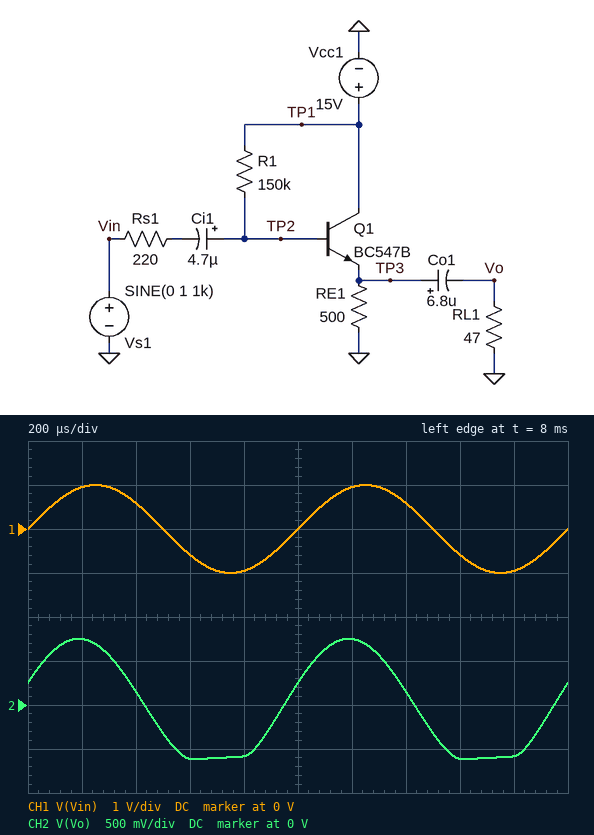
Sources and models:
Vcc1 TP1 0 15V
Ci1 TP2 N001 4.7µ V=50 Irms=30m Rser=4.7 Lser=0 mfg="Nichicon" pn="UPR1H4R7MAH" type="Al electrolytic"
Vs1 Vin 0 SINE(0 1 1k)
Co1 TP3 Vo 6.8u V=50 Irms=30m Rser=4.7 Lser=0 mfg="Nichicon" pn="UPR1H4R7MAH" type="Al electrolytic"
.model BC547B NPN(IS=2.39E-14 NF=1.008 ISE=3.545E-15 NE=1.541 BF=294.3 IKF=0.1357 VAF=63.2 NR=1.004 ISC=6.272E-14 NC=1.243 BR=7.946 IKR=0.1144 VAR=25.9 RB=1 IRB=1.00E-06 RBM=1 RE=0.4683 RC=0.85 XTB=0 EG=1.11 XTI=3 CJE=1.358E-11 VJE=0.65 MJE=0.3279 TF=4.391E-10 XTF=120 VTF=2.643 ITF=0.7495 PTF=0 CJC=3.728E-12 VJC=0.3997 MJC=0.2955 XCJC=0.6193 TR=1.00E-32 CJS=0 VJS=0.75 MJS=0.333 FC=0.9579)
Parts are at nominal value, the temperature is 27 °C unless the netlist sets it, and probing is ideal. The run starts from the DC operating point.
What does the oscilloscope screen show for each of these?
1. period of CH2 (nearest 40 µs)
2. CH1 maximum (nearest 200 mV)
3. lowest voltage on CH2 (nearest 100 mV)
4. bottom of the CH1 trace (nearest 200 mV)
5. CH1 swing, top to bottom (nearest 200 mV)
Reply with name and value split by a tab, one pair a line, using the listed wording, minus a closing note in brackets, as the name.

period of CH2	1.00 ms
CH1 maximum	1.0 V
lowest voltage on CH2	-600 mV
bottom of the CH1 trace	-1.0 V
CH1 swing, top to bottom	2.0 V
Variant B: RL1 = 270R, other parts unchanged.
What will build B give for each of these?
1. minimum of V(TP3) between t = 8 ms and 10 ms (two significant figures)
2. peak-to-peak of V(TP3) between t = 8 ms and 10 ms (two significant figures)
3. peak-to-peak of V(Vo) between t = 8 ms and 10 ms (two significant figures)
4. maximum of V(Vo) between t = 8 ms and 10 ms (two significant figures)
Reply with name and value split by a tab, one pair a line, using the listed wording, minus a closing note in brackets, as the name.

minimum of V(TP3) between t = 8 ms and 10 ms	6.1 V
peak-to-peak of V(TP3) between t = 8 ms and 10 ms	2.0 V
peak-to-peak of V(Vo) between t = 8 ms and 10 ms	1.9 V
maximum of V(Vo) between t = 8 ms and 10 ms	960 mV
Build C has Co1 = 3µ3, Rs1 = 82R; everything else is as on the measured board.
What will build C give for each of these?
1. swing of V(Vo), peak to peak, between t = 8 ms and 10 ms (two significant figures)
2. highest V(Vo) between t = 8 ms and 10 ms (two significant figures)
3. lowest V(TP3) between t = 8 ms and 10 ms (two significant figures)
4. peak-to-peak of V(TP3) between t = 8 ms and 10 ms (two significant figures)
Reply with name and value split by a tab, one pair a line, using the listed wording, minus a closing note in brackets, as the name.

swing of V(Vo), peak to peak, between t = 8 ms and 10 ms	1.2 V
highest V(Vo) between t = 8 ms and 10 ms	640 mV
lowest V(TP3) between t = 8 ms and 10 ms	6.1 V
peak-to-peak of V(TP3) between t = 8 ms and 10 ms	1.9 V
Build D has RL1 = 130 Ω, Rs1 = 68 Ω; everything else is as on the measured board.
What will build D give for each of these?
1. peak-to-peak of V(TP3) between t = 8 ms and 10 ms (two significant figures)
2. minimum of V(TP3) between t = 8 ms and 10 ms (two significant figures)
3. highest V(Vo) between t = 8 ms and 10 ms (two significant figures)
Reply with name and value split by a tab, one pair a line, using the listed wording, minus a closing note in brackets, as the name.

peak-to-peak of V(TP3) between t = 8 ms and 10 ms	1.9 V
minimum of V(TP3) between t = 8 ms and 10 ms	6.1 V
highest V(Vo) between t = 8 ms and 10 ms	930 mV
